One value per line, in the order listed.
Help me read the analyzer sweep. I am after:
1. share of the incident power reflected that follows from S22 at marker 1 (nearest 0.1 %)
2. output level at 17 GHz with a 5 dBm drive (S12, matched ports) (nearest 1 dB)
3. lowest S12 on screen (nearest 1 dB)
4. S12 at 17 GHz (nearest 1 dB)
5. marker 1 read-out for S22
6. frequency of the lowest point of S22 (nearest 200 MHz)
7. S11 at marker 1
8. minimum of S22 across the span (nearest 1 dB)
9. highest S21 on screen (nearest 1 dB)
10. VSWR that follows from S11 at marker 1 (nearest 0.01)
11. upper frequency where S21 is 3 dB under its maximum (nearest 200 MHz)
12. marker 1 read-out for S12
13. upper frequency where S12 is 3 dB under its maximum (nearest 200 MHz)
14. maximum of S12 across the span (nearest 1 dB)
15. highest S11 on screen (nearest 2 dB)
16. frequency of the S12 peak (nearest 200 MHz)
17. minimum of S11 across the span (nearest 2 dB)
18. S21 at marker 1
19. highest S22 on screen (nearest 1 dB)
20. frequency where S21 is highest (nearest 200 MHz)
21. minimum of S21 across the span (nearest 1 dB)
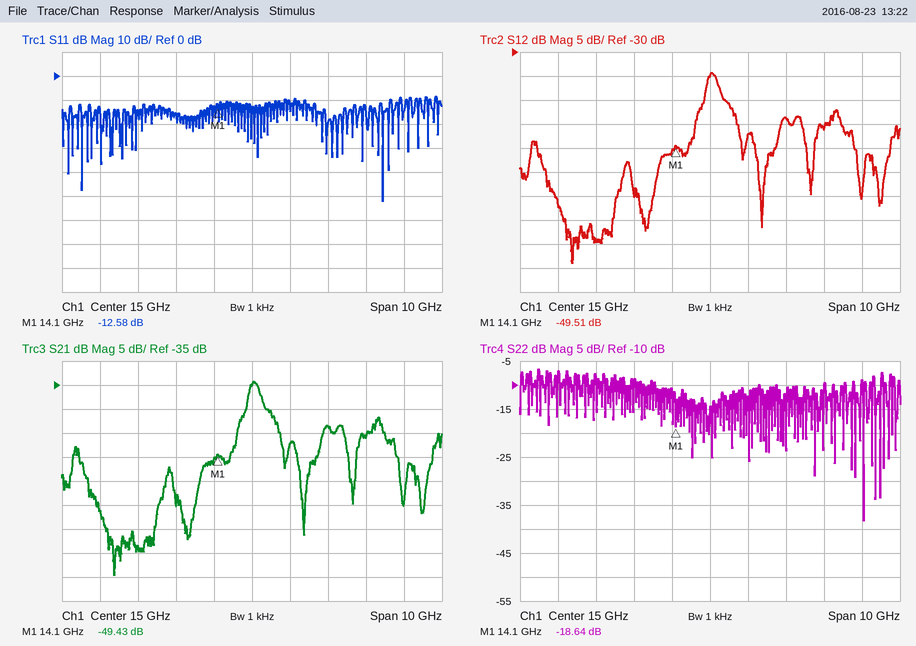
1.4 %
-39 dBm
-74 dB
-44 dB
-18.64 dB
19.0 GHz
-12.58 dB
-38 dB
-34 dB
1.61
15.2 GHz
-49.51 dB
15.2 GHz
-34 dB
-8 dB
15.0 GHz
-52 dB
-49.43 dB
-7 dB
15.0 GHz
-75 dB
